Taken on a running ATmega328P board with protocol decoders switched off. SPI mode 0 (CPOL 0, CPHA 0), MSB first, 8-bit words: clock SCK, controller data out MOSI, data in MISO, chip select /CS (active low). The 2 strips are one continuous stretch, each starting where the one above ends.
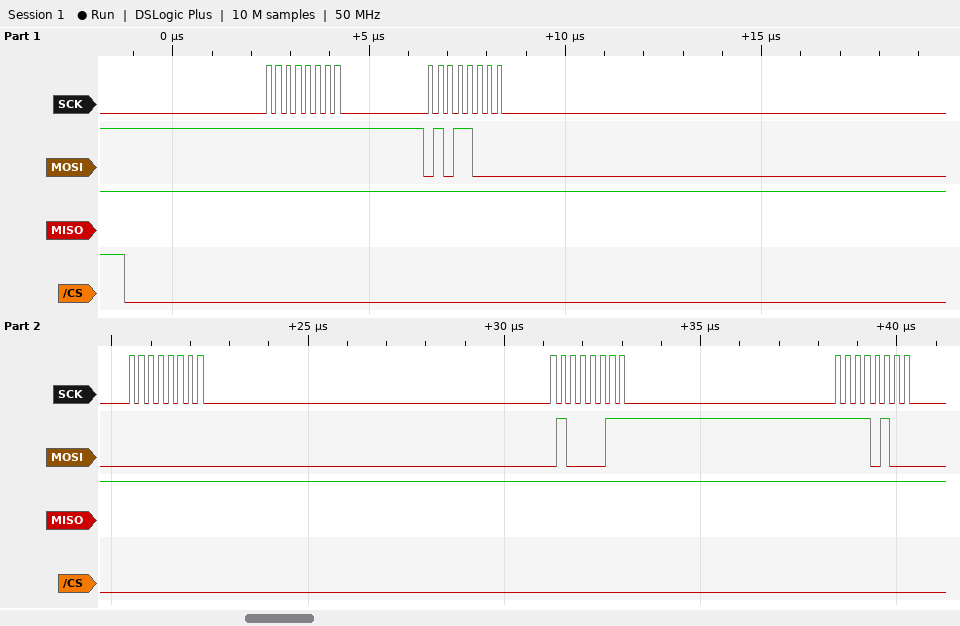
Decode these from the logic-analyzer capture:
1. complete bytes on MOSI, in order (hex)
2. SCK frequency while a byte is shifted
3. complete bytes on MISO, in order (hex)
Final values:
0xFF 0x58 0x00 0x43 0xF4
4 MHz
0xFF 0xFF 0xFF 0xFF 0xFF
